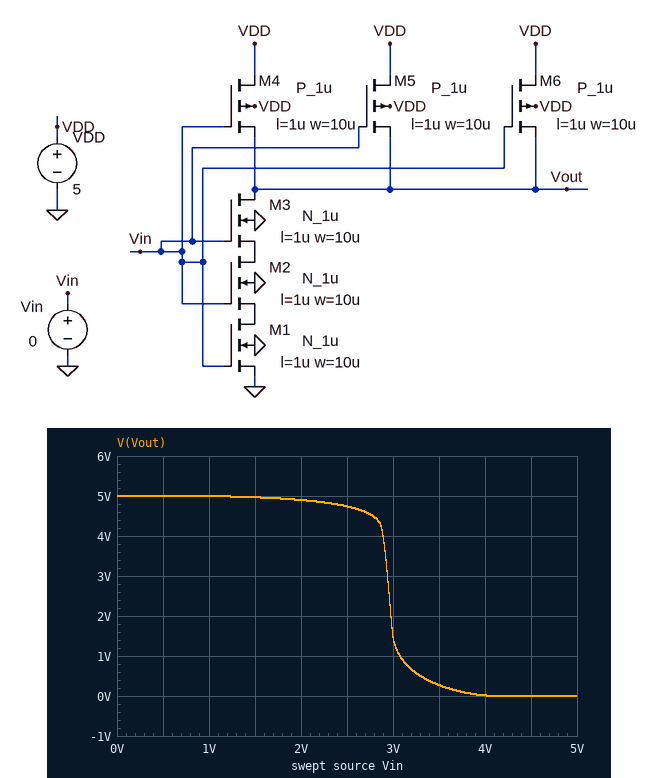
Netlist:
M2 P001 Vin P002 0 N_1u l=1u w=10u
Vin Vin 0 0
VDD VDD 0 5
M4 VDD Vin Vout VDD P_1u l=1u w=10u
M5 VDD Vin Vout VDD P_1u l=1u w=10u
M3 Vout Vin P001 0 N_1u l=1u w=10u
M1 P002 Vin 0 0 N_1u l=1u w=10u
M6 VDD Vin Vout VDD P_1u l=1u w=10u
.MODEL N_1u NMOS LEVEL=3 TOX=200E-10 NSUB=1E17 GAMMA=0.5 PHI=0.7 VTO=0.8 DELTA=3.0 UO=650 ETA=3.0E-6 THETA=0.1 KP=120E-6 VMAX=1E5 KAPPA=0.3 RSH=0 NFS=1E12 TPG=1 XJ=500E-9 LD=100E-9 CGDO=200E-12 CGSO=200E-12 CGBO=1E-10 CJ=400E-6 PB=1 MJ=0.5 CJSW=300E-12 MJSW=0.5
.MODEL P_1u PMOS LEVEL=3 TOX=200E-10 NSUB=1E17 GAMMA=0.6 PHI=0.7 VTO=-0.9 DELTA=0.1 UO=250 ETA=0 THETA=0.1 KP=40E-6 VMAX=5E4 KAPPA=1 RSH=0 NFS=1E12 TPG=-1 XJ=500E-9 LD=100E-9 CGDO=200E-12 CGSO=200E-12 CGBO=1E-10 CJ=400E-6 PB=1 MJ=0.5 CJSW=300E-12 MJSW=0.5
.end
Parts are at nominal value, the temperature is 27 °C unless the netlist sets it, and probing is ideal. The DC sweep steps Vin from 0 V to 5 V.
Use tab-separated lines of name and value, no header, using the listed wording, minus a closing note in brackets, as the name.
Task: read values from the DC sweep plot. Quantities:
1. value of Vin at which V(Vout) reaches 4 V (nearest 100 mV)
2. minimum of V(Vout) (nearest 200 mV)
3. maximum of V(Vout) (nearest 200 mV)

value of Vin at which V(Vout) reaches 4 V	2.9 V
minimum of V(Vout)	0 V
maximum of V(Vout)	5.0 V
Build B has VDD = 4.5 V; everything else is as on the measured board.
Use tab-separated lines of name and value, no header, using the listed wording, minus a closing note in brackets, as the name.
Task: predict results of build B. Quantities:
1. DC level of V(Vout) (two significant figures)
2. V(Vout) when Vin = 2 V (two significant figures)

DC level of V(Vout)	4.5 V
V(Vout) when Vin = 2 V	4.4 V
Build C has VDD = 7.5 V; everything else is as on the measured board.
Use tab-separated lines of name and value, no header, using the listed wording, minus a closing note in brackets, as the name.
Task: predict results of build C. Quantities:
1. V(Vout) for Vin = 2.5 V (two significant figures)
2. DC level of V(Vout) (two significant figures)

V(Vout) for Vin = 2.5 V	7.4 V
DC level of V(Vout)	7.5 V
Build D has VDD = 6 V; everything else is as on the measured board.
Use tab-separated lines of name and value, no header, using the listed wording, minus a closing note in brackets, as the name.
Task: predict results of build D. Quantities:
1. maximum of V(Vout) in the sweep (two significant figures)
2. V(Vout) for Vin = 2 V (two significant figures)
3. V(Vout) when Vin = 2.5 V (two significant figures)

maximum of V(Vout) in the sweep	6.0 V
V(Vout) for Vin = 2 V	5.9 V
V(Vout) when Vin = 2.5 V	5.8 V
